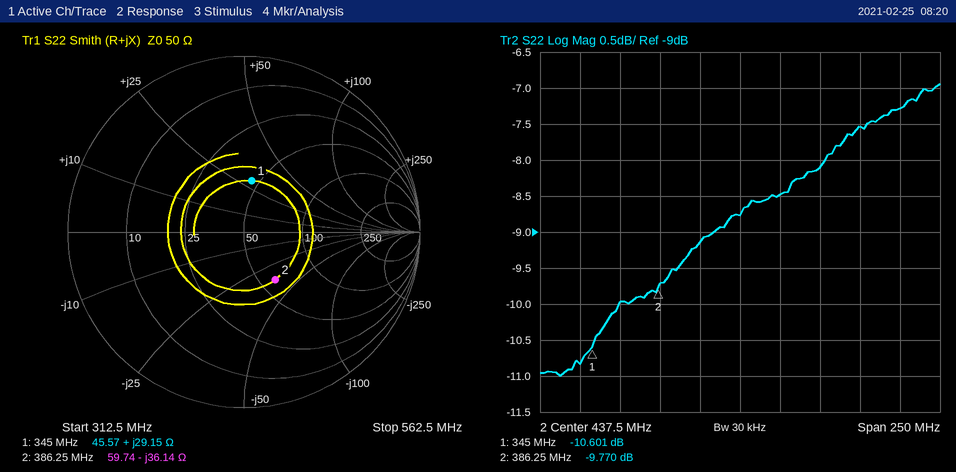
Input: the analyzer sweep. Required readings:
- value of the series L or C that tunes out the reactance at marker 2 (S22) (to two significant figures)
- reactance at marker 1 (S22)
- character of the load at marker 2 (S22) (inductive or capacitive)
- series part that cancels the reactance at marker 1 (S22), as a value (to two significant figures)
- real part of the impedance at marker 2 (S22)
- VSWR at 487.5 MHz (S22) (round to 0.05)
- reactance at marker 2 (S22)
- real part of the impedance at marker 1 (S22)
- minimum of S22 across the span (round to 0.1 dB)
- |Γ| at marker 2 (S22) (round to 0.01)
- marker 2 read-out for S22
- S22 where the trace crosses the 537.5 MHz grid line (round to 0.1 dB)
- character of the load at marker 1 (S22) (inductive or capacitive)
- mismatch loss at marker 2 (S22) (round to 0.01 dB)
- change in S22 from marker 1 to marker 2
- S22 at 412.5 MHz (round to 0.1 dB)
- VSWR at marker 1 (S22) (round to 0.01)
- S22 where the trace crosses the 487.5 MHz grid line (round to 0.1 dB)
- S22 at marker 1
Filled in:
15 nH
+29.15 Ω
capacitive
16 pF
59.74 Ω
2.30
-36.14 Ω
45.57 Ω
-11.0 dB
0.32
-9.770 dB
-7.3 dB
inductive
0.48 dB
0.831 dB
-9.1 dB
1.84
-8.1 dB
-10.601 dB
